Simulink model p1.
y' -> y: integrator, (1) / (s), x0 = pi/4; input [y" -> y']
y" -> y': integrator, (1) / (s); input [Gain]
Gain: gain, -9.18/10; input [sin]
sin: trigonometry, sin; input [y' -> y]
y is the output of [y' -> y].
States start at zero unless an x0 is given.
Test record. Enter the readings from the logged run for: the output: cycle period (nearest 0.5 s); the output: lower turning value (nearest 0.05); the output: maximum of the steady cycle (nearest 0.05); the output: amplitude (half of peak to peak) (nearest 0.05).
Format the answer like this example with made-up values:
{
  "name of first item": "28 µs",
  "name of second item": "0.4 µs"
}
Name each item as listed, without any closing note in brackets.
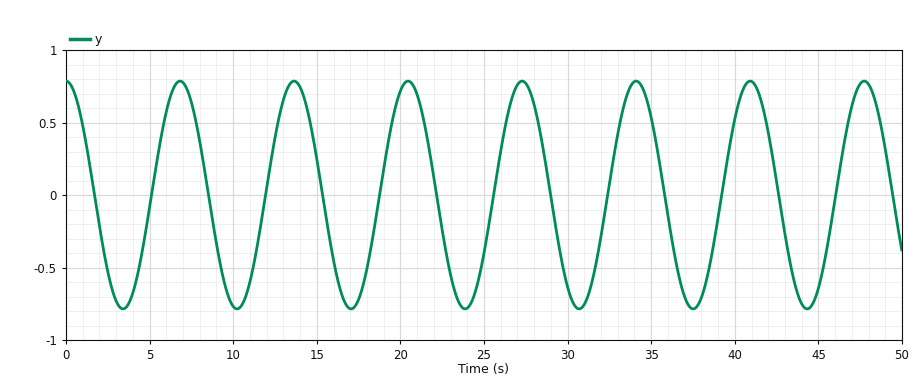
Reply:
{
  "the output: cycle period": "7.0 s",
  "the output: lower turning value": "-0.80",
  "the output: maximum of the steady cycle": "0.80",
  "the output: amplitude (half of peak to peak)": "0.80"
}
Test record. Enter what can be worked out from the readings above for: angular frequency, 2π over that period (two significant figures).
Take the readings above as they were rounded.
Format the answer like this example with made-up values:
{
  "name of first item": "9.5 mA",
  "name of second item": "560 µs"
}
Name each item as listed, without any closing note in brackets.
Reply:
{
  "angular frequency, 2π over that period": "0.90 rad/s"
}
